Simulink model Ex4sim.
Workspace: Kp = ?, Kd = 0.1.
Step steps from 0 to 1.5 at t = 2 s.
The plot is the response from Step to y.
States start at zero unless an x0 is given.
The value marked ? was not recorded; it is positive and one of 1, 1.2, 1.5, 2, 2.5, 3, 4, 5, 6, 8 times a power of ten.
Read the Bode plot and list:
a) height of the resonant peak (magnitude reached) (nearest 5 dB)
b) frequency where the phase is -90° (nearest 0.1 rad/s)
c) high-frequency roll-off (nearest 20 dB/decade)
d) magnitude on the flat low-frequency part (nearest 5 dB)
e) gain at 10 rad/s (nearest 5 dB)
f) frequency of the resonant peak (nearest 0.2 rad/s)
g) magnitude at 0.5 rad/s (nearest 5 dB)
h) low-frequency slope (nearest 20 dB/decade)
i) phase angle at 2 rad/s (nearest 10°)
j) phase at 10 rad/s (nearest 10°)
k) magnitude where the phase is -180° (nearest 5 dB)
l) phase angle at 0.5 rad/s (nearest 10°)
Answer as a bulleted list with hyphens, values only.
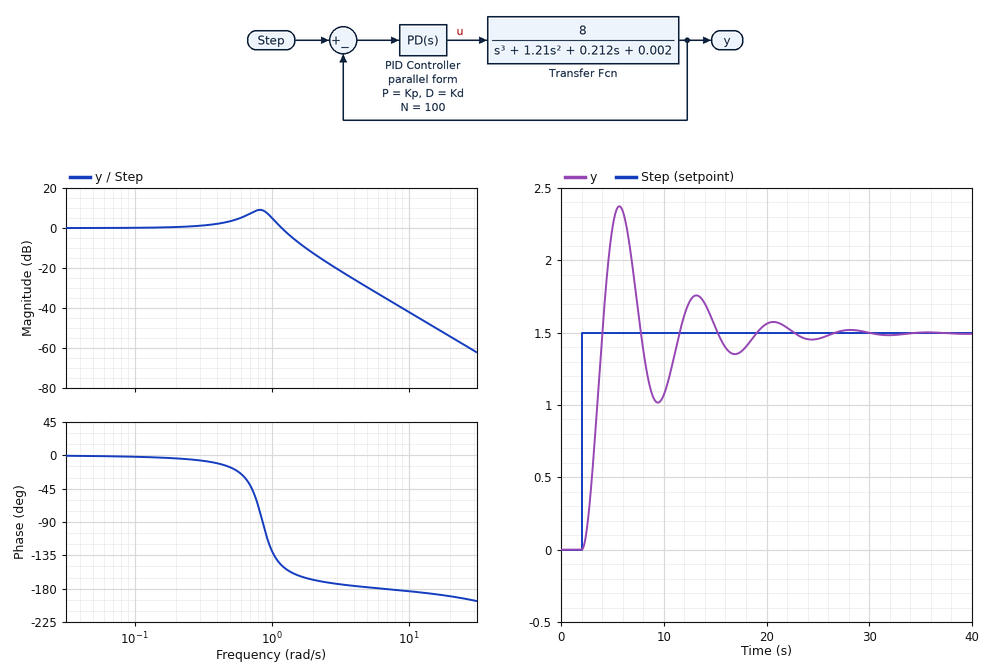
- 10 dB
- 0.9 rad/s
- -40 dB/decade
- 0 dB
- -40 dB
- 0.8 rad/s
- 5 dB
- 0 dB/decade
- -170°
- -180°
- -35 dB
- -20°
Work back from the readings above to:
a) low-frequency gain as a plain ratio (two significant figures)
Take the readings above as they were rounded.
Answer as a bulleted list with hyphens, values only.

- 1.0
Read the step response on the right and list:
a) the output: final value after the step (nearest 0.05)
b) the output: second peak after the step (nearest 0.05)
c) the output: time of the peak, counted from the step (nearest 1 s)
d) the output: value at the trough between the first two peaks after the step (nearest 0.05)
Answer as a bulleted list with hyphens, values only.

- 1.50
- 1.75
- 4 s
- 1.00
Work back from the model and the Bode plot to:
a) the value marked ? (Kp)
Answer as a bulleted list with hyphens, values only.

- 0.08
